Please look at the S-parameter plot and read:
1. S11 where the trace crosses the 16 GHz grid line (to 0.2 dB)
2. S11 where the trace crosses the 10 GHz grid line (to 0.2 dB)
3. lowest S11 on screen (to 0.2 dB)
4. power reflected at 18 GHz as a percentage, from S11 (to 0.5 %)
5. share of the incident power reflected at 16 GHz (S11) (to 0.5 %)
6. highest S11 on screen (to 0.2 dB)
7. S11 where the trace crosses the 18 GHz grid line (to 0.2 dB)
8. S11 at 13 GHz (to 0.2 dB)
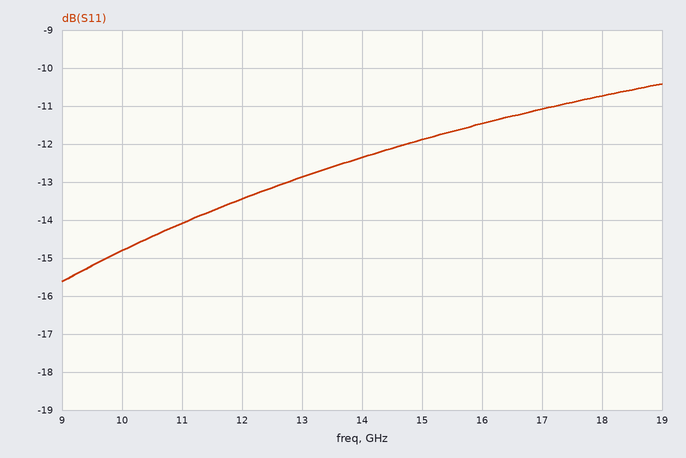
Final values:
-11.4 dB
-14.8 dB
-15.6 dB
8.5 %
7.0 %
-10.4 dB
-10.8 dB
-12.8 dB
